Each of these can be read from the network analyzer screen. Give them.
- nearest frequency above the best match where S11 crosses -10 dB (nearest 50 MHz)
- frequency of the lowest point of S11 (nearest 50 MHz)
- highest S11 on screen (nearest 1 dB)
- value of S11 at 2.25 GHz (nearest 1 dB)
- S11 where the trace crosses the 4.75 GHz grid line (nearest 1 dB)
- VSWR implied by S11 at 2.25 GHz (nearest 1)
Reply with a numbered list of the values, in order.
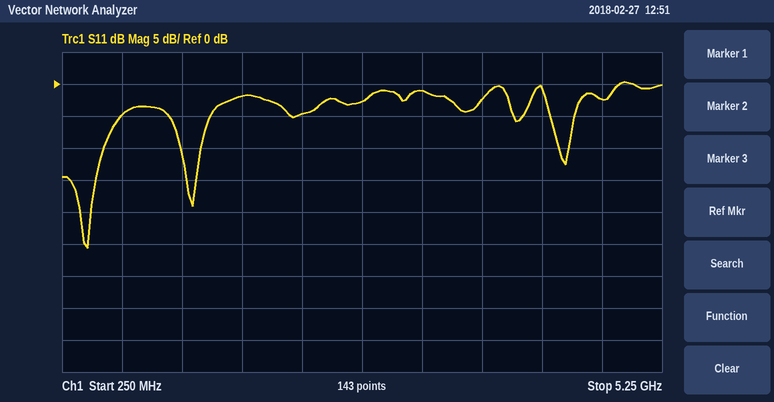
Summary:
1. 600 MHz
2. 450 MHz
3. 0 dB
4. -5 dB
5. -2 dB
6. 4
